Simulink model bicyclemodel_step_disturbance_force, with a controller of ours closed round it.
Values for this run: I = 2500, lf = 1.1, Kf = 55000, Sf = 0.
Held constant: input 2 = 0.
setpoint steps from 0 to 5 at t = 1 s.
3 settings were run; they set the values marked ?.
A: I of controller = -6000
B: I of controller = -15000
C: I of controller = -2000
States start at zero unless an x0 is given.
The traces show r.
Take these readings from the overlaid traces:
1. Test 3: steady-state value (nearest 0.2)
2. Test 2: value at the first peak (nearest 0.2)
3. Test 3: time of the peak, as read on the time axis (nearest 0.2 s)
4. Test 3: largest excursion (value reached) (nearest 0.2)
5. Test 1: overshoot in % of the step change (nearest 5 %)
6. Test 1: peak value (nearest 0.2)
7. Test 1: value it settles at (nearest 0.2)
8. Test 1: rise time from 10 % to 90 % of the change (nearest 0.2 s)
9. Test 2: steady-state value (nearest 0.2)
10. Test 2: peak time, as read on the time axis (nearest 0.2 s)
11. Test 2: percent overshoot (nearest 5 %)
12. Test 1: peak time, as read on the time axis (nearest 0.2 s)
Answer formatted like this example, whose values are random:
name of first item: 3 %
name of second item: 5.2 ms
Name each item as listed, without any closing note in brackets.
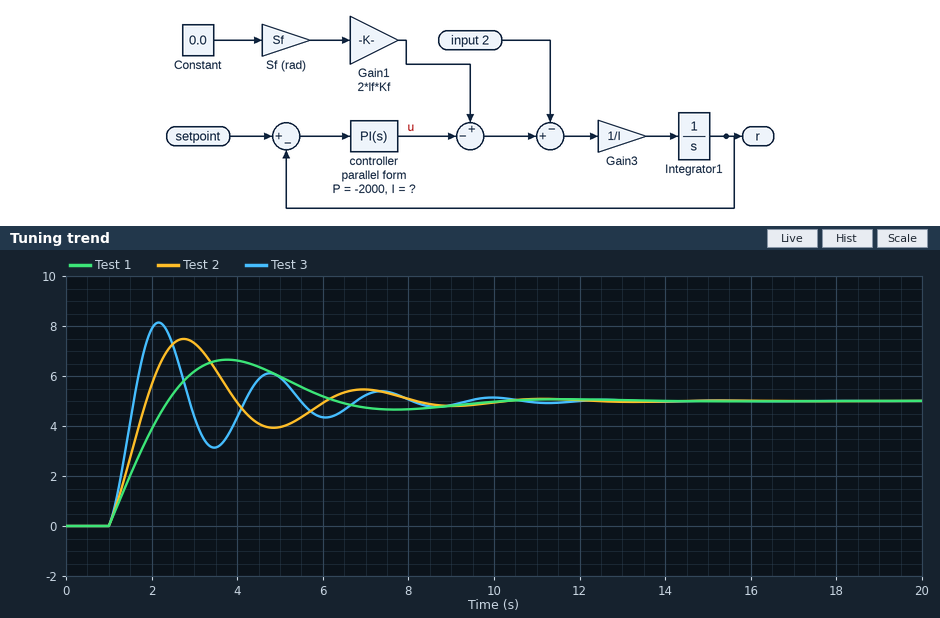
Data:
Test 3: steady-state value: 5.0
Test 2: value at the first peak: 7.4
Test 3: time of the peak, as read on the time axis: 2.2 s
Test 3: largest excursion (value reached): 8.2
Test 1: overshoot in % of the step change: 35 %
Test 1: peak value: 6.6
Test 1: value it settles at: 5.0
Test 1: rise time from 10 % to 90 % of the change: 1.0 s
Test 2: steady-state value: 5.0
Test 2: peak time, as read on the time axis: 2.8 s
Test 2: percent overshoot: 50 %
Test 1: peak time, as read on the time axis: 3.8 s
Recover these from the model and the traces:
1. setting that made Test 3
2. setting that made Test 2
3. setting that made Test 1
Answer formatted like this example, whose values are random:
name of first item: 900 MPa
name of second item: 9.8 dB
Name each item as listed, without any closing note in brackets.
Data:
setting that made Test 3: B
setting that made Test 2: A
setting that made Test 1: C
